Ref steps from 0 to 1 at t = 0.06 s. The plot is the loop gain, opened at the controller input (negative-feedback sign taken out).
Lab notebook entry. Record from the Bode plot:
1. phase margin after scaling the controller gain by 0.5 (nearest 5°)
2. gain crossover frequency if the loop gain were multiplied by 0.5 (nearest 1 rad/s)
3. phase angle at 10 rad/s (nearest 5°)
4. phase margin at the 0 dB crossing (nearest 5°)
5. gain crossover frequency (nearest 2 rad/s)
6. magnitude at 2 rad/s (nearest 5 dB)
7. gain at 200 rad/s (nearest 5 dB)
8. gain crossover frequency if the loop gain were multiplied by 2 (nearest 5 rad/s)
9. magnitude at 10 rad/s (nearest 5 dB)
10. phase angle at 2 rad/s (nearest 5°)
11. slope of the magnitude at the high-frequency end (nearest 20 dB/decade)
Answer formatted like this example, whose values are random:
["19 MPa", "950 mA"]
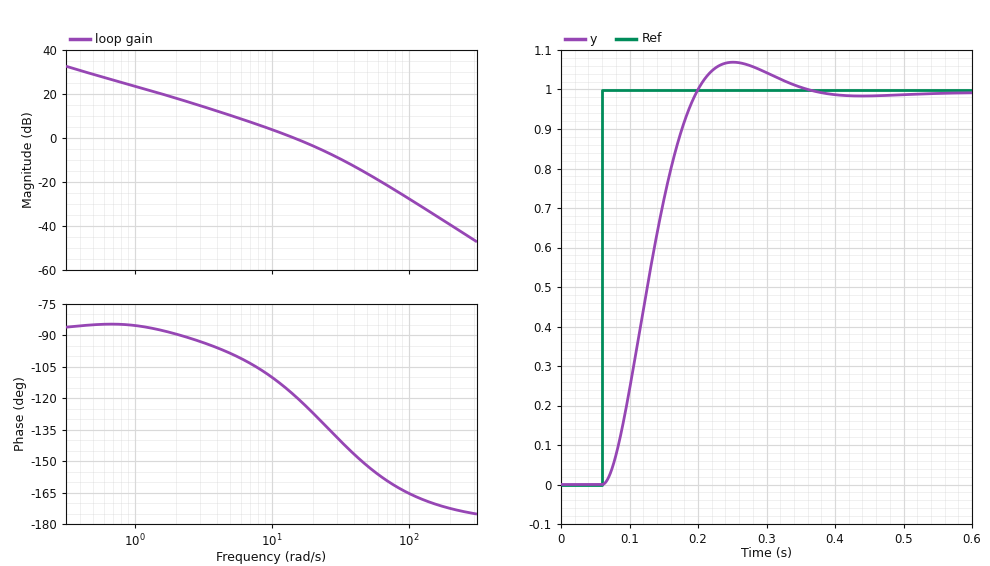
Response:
["75°", "8 rad/s", "-110°", "60°", "14 rad/s", "20 dB", "-40 dB", "25 rad/s", "5 dB", "-90°", "-40 dB/decade"]
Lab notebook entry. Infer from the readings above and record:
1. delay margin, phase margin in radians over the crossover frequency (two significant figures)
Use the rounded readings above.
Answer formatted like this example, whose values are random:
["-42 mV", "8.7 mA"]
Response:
["0.075 s"]
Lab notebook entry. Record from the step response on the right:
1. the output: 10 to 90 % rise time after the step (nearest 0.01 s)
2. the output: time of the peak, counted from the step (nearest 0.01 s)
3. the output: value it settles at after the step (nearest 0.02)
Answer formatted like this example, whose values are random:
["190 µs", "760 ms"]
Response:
["0.09 s", "0.19 s", "1.00"]
